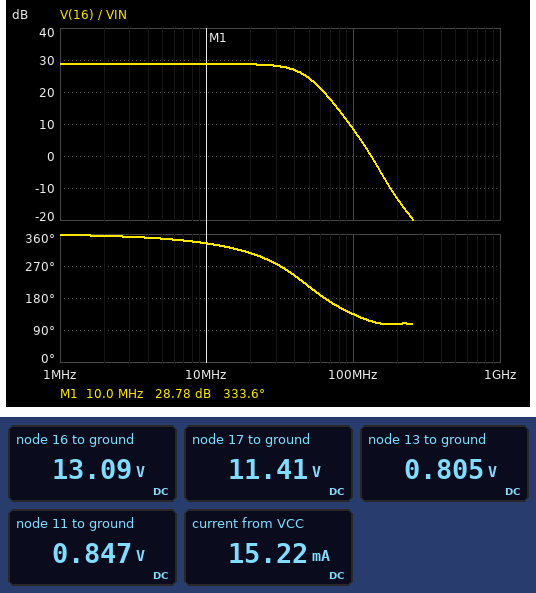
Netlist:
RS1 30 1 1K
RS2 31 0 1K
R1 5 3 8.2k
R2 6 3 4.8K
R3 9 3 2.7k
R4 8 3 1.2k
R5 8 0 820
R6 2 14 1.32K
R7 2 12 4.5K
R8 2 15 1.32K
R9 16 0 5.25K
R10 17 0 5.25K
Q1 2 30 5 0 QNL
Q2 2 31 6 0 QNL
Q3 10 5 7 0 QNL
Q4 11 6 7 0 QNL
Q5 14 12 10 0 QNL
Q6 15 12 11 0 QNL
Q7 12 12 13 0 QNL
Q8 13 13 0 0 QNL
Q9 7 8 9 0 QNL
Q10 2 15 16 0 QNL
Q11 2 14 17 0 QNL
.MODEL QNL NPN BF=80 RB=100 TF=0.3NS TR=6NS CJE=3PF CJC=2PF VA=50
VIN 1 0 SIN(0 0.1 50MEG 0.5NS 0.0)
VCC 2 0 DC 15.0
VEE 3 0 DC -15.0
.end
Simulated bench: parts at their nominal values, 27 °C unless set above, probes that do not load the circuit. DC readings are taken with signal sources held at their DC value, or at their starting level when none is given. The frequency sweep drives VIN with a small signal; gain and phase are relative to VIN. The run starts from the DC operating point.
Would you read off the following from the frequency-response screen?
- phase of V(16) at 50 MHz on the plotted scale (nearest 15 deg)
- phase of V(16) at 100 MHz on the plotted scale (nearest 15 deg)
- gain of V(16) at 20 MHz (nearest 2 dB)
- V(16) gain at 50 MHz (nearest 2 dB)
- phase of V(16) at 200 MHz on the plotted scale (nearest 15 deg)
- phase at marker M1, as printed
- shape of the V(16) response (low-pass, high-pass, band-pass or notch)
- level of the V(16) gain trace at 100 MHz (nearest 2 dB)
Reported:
210 deg
135 deg
28 dB
24 dB
105 deg
333.6 deg
low-pass
8 dB
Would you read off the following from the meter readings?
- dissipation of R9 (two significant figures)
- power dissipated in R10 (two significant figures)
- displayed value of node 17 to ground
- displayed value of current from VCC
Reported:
33 mW
25 mW
11.41 V
15.22 mA
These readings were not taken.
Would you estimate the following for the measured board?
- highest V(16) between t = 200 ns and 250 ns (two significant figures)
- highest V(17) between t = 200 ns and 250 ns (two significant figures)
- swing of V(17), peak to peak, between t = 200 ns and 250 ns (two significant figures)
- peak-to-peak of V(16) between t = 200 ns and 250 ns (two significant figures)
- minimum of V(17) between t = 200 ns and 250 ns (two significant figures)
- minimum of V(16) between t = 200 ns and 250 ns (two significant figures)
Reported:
14 V
13 V
2.7 V
2.6 V
11 V
11 V
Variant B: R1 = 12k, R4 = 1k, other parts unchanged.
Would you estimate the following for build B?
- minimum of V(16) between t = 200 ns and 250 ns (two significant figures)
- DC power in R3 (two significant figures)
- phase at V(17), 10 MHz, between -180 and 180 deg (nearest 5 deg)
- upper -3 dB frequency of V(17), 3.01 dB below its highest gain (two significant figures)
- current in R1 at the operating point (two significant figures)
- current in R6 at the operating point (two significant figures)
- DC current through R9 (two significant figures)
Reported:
12 V
20 mW
160 deg
52 MHz
1.2 mA
2.2 mA
2.6 mA
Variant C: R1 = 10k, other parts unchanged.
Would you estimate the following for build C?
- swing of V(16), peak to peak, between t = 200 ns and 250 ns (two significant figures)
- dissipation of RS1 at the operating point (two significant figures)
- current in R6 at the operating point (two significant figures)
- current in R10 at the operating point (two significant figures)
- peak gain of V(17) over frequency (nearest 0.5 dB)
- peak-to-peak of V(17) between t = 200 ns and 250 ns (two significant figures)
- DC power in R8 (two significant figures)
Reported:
2.5 V
190 nW
2.3 mA
2.1 mA
27.5 dB
2.6 V
600 µW
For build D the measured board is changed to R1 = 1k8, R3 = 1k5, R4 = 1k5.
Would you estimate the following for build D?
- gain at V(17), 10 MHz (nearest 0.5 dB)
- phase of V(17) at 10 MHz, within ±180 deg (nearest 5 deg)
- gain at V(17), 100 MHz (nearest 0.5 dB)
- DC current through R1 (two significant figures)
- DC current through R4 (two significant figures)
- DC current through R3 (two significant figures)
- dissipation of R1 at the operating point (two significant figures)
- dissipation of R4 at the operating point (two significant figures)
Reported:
24.5 dB
155 deg
7.0 dB
7.8 mA
6.4 mA
5.9 mA
110 mW
62 mW
